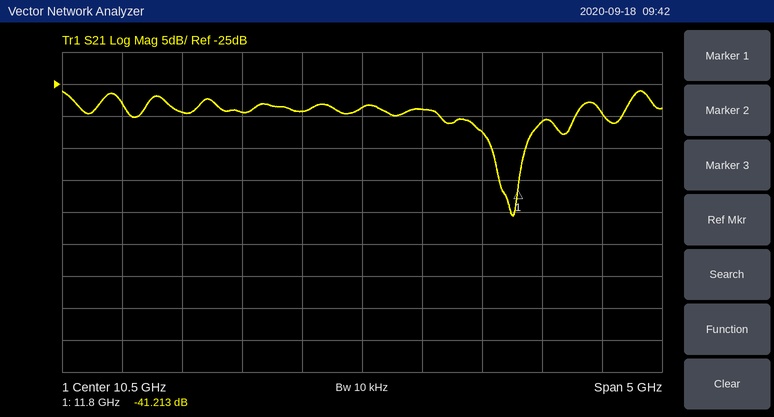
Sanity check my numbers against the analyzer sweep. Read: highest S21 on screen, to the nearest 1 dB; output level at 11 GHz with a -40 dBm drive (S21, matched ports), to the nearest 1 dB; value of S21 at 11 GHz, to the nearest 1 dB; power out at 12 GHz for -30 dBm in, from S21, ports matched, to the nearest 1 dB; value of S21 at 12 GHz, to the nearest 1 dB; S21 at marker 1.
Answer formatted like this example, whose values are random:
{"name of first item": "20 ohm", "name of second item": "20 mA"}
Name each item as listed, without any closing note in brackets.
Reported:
{"highest S21 on screen, to the nearest 1 dB": "-26 dB", "output level at 11 GHz with a -40 dBm drive (S21, matched ports), to the nearest 1 dB": "-69 dBm", "value of S21 at 11 GHz, to the nearest 1 dB": "-29 dB", "power out at 12 GHz for -30 dBm in, from S21, ports matched, to the nearest 1 dB": "-61 dBm", "value of S21 at 12 GHz, to the nearest 1 dB": "-31 dB", "S21 at marker 1": "-41.213 dB"}
